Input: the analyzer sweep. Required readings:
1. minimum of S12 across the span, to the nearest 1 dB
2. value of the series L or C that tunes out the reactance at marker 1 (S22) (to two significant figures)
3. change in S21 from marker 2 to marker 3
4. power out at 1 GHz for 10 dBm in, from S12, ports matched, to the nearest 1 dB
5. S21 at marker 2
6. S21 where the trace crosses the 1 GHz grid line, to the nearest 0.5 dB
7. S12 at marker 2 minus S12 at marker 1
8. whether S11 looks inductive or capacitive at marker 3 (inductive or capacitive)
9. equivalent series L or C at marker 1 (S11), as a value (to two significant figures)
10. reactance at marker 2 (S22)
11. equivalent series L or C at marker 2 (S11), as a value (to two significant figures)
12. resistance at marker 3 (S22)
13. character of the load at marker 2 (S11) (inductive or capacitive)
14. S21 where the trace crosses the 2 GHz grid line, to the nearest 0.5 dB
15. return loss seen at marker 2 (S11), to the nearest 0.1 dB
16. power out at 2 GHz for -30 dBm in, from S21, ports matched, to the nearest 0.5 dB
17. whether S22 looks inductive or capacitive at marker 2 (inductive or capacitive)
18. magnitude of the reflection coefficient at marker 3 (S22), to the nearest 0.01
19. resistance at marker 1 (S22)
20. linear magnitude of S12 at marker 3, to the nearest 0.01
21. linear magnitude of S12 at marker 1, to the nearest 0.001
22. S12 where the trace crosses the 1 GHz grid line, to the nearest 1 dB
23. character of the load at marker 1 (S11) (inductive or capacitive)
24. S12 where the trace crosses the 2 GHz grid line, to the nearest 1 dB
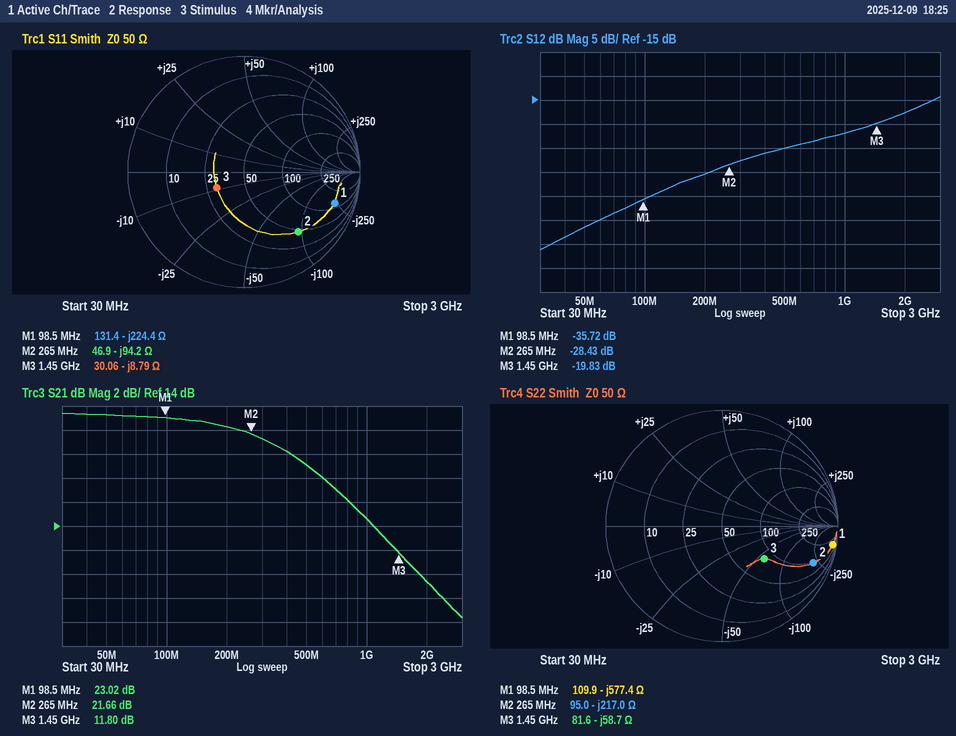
-46 dB
930 nH
-9.86 dB
-12 dBm
21.66 dB
14.5 dB
7.29 dB
capacitive
7.2 pF
-217.0 Ω
6.4 pF
81.6 Ω
capacitive
9.5 dB
3.1 dB
-20.5 dBm
capacitive
0.46
109.9 Ω
0.10
0.016
-22 dB
capacitive
-18 dB
